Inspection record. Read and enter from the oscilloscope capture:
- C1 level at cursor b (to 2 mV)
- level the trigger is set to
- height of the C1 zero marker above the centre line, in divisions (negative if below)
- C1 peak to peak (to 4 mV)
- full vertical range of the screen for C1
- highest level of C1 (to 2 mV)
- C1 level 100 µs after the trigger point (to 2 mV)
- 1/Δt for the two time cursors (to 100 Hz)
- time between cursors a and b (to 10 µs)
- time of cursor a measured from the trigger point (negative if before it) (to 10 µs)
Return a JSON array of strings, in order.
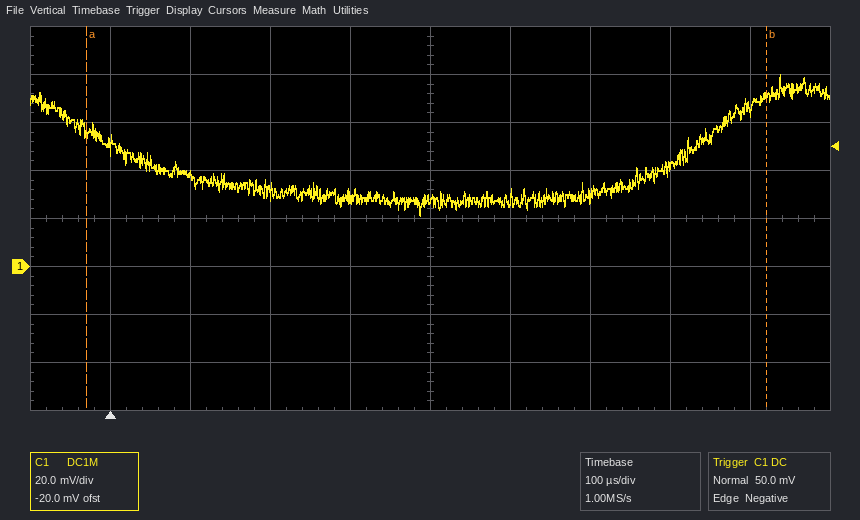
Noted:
["70 mV", "50.0 mV", "-1.0 div", "60 mV", "160 mV", "80 mV", "38 mV", "1.2 kHz", "850 µs", "-30 µs"]
